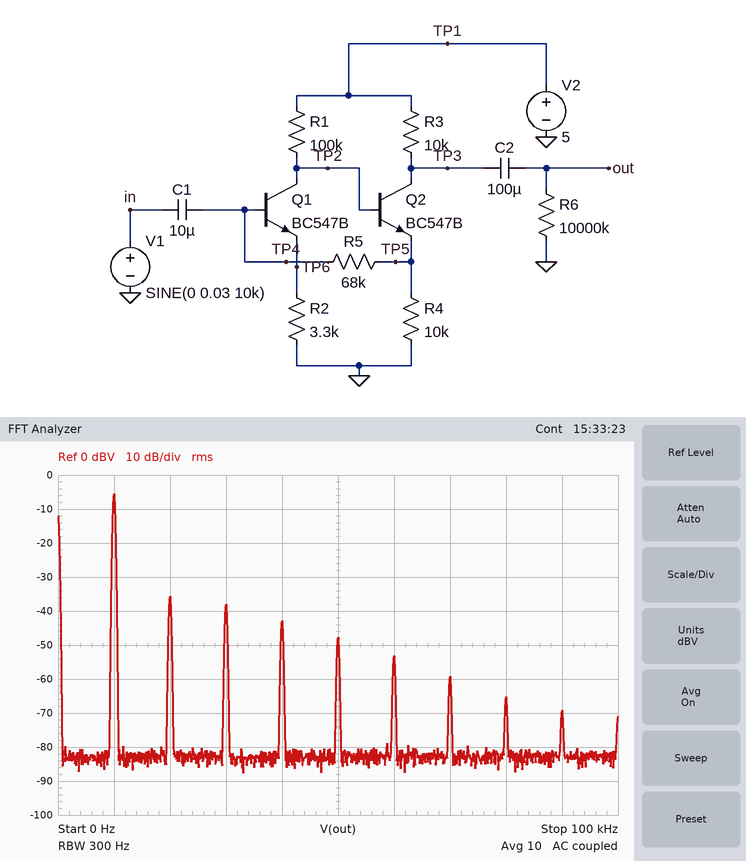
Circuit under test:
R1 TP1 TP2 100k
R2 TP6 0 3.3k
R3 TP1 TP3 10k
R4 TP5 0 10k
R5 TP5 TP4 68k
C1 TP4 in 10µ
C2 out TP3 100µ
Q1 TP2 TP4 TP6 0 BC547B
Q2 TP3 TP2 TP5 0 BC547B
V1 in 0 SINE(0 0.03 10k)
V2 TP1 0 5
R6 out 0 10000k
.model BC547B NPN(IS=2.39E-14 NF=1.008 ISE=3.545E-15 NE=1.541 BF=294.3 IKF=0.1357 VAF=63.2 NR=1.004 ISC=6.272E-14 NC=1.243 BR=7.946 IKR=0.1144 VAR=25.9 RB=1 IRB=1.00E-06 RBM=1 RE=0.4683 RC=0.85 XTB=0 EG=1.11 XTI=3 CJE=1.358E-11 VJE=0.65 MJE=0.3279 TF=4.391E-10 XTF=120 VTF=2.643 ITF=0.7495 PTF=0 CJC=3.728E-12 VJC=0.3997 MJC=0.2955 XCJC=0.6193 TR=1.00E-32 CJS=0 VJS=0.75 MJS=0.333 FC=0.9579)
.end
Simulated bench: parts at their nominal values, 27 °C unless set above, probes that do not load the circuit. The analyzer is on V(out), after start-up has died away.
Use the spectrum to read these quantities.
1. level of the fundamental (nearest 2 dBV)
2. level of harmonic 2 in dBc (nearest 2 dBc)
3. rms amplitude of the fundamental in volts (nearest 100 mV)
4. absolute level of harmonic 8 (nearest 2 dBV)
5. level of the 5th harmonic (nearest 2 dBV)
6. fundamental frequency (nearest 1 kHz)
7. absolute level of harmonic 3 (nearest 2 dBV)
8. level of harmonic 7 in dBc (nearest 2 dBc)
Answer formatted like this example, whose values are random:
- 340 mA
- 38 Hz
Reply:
- -6 dBV
- -30 dBc
- 500 mV
- -66 dBV
- -48 dBV
- 10 kHz
- -38 dBV
- -54 dBc
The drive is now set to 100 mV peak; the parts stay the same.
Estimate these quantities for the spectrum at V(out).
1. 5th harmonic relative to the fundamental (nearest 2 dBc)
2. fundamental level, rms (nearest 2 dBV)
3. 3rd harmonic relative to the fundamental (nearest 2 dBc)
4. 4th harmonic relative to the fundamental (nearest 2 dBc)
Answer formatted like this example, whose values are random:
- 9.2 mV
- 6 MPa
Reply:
- -32 dBc
- 0 dBV
- -16 dBc
- -20 dBc
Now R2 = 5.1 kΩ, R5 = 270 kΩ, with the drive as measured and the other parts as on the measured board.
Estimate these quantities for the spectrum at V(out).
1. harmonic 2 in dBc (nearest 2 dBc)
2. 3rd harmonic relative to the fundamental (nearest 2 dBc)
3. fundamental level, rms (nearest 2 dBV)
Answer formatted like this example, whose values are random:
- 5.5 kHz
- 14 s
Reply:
- -50 dBc
- -54 dBc
- -10 dBV
